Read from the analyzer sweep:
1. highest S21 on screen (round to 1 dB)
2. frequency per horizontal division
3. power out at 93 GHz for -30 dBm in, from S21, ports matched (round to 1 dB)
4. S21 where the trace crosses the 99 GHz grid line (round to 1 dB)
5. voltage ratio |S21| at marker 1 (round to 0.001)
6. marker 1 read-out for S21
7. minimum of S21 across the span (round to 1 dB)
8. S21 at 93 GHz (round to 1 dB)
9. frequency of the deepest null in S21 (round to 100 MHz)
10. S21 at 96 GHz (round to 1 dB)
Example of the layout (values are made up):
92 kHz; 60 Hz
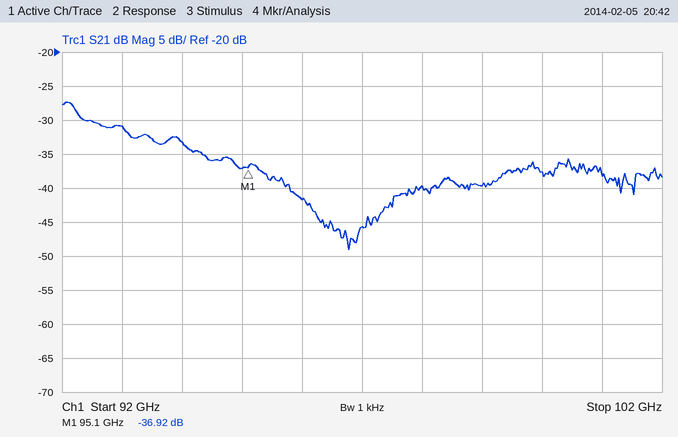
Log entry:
-27 dB; 1 GHz; -61 dBm; -40 dB; 0.014; -36.92 dB; -49 dB; -31 dB; 96.8 GHz; -42 dB
